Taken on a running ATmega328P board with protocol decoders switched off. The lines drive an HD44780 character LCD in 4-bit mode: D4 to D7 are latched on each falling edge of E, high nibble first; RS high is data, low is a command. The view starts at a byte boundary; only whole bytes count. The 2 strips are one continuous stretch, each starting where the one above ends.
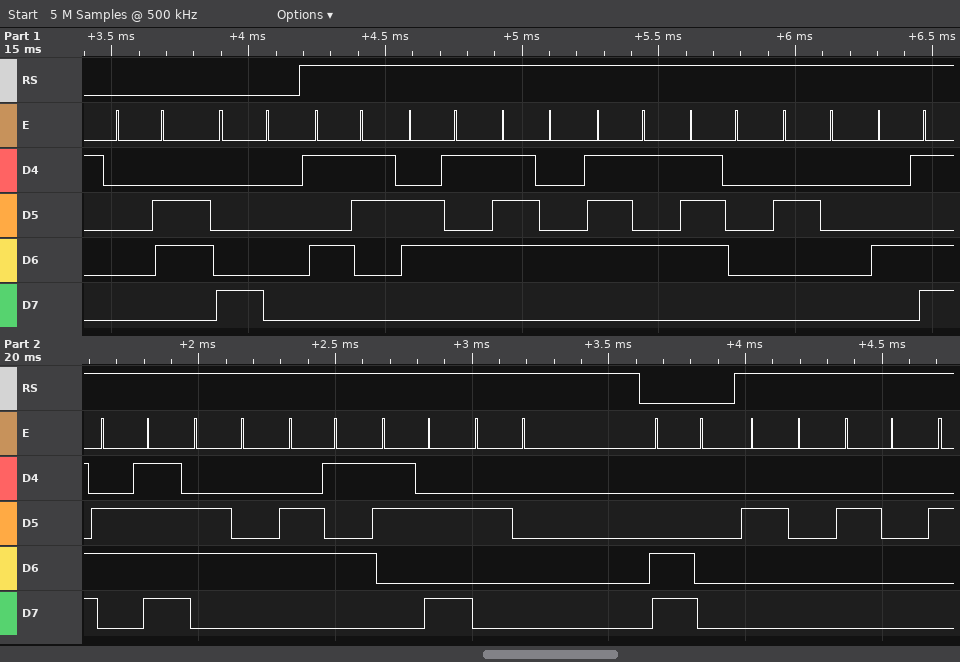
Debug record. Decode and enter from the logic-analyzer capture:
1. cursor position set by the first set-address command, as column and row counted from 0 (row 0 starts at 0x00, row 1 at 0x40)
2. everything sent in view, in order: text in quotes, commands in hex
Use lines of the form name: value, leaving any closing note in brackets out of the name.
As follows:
cursor position set by the first set-address command, as column and row counted from 0: column 0, row 0
everything sent in view, in order: text in quotes, commands in hex: 0x06 0x80 "Setup Mode: " 0xC0 "  "
